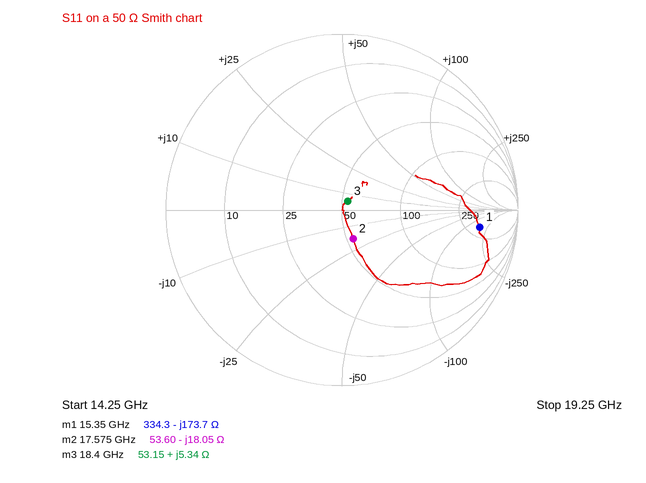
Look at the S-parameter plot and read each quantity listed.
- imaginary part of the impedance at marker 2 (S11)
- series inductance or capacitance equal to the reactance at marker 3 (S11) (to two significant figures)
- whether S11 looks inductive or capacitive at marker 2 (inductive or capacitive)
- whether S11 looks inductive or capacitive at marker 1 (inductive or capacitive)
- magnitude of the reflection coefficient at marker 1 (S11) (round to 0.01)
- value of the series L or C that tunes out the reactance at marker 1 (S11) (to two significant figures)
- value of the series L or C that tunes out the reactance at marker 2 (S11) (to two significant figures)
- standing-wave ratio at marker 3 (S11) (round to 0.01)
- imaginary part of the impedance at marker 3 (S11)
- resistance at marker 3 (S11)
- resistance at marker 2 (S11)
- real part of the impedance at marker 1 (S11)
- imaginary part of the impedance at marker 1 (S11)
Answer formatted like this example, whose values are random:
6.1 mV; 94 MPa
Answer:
-18.05 Ω; 46 pH; capacitive; capacitive; 0.79; 1.8 nH; 160 pH; 1.13; +5.34 Ω; 53.15 Ω; 53.60 Ω; 334.3 Ω; -173.7 Ω
